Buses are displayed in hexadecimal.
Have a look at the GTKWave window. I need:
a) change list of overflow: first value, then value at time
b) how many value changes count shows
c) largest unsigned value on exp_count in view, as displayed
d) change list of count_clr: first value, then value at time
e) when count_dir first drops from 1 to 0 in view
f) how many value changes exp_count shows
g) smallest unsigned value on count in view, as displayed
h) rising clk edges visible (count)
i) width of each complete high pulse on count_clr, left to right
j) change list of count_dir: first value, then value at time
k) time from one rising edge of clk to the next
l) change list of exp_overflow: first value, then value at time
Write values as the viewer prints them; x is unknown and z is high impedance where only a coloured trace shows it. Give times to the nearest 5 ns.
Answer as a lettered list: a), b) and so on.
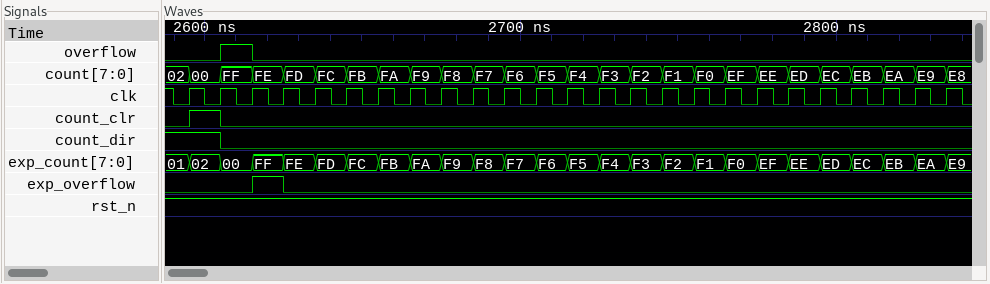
a) 0, 1 at 2605 ns, 0 at 2615 ns
b) 25
c) FF
d) 0, 1 at 2595 ns, 0 at 2605 ns
e) 2605 ns
f) 25
g) 00
h) 25
i) 10 ns
j) 1, 0 at 2605 ns
k) 10 ns
l) 0, 1 at 2615 ns, 0 at 2625 ns
